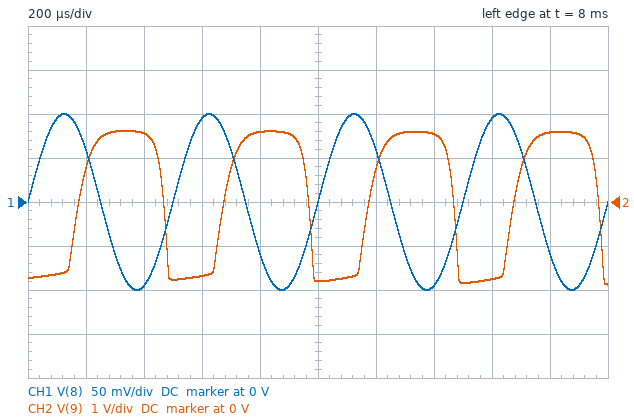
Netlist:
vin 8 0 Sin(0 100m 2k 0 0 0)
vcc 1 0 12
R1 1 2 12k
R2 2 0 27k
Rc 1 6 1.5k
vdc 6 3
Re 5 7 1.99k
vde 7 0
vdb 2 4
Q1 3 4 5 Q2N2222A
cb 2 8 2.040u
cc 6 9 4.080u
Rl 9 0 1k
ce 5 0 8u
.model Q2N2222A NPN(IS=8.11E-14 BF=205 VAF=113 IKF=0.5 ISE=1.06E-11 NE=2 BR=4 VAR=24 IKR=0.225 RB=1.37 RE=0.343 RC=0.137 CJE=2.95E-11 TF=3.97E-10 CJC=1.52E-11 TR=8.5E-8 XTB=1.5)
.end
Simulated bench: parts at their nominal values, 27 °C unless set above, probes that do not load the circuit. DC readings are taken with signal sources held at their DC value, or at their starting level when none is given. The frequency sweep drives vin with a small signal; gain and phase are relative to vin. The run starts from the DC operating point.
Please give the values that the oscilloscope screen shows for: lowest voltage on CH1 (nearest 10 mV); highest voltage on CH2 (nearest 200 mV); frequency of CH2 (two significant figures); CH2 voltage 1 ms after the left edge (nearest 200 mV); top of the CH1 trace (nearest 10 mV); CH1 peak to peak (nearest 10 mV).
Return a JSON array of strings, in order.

["-100 mV", "1.6 V", "2.0 kHz", "-1.8 V", "100 mV", "200 mV"]
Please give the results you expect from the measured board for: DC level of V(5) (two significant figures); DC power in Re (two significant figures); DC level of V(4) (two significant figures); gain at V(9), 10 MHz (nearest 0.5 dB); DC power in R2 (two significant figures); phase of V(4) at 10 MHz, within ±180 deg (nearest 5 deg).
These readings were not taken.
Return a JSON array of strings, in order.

["6.9 V", "24 mW", "7.5 V", "5.0 dB", "2.1 mW", "0 deg"]
